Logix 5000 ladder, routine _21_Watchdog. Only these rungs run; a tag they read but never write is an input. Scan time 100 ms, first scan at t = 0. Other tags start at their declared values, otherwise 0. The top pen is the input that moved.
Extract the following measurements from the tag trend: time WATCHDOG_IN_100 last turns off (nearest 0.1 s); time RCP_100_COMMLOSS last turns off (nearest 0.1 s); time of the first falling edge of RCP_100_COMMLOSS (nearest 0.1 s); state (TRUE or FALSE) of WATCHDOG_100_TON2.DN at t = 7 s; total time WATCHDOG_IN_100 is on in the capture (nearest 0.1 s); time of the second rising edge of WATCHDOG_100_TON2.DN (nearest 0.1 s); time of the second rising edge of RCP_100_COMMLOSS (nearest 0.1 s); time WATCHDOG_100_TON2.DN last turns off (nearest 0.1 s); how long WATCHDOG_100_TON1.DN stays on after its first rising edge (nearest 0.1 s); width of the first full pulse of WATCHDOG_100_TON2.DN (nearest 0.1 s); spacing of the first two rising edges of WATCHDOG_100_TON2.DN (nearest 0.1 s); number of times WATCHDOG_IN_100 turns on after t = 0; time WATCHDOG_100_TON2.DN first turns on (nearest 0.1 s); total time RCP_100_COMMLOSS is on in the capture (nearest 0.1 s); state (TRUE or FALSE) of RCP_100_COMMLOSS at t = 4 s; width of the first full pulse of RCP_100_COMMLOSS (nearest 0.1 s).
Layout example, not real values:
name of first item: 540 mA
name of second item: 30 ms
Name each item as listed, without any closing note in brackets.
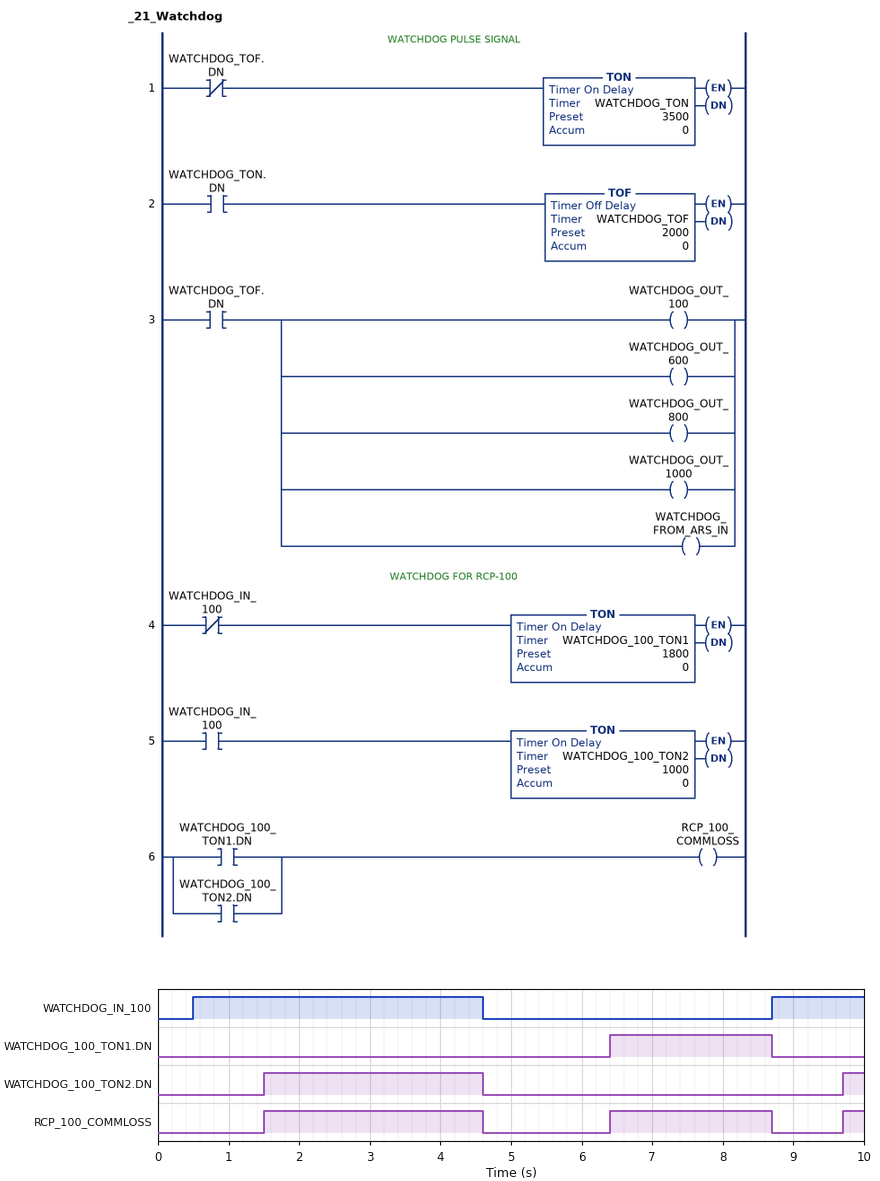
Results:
time WATCHDOG_IN_100 last turns off: 4.6 s
time RCP_100_COMMLOSS last turns off: 8.7 s
time of the first falling edge of RCP_100_COMMLOSS: 4.6 s
state (TRUE or FALSE) of WATCHDOG_100_TON2.DN at t = 7 s: FALSE
total time WATCHDOG_IN_100 is on in the capture: 5.4 s
time of the second rising edge of WATCHDOG_100_TON2.DN: 9.7 s
time of the second rising edge of RCP_100_COMMLOSS: 6.4 s
time WATCHDOG_100_TON2.DN last turns off: 4.6 s
how long WATCHDOG_100_TON1.DN stays on after its first rising edge: 2.3 s
width of the first full pulse of WATCHDOG_100_TON2.DN: 3.1 s
spacing of the first two rising edges of WATCHDOG_100_TON2.DN: 8.2 s
number of times WATCHDOG_IN_100 turns on after t = 0: 2
time WATCHDOG_100_TON2.DN first turns on: 1.5 s
total time RCP_100_COMMLOSS is on in the capture: 5.7 s
state (TRUE or FALSE) of RCP_100_COMMLOSS at t = 4 s: TRUE
width of the first full pulse of RCP_100_COMMLOSS: 3.1 s
